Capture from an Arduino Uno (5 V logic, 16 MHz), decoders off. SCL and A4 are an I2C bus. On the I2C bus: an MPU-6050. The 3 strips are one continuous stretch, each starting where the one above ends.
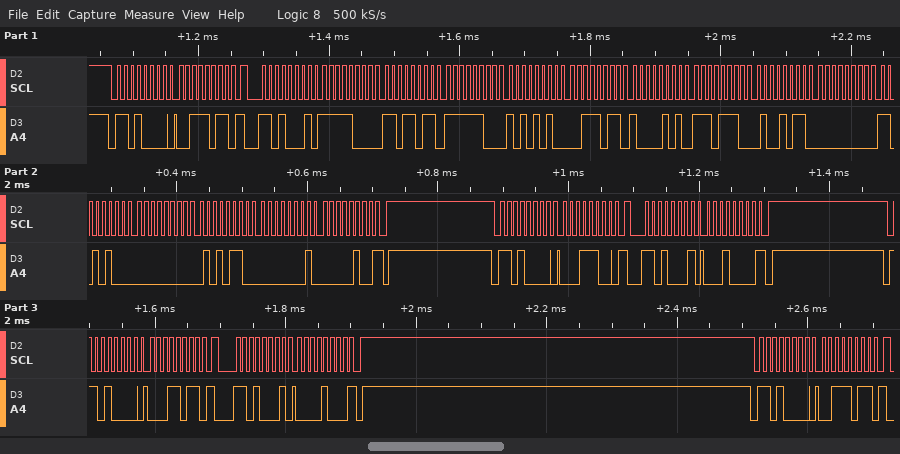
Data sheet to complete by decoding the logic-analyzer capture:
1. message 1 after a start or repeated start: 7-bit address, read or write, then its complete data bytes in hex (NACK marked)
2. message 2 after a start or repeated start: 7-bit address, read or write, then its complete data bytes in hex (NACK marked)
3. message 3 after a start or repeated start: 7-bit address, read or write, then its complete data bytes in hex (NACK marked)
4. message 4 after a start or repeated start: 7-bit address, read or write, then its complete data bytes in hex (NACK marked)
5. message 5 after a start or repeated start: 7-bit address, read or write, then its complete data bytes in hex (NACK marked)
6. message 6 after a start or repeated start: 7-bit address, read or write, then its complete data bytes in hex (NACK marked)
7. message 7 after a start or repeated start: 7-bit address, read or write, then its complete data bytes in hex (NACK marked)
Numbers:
0x68 write: 3B
0x68 read: F8 DB FC AA 3B 85 EE 4B 00 D4 00 56 01 04 NACK
0x68 write: 1C
0x68 read: 10 NACK
0x68 write: 1B
0x68 read: 08 NACK
0x68 write: 3B
